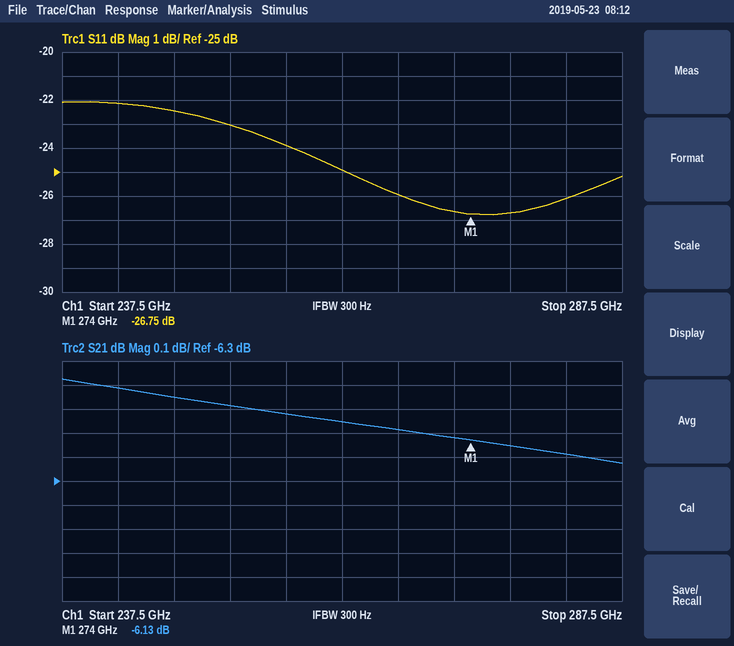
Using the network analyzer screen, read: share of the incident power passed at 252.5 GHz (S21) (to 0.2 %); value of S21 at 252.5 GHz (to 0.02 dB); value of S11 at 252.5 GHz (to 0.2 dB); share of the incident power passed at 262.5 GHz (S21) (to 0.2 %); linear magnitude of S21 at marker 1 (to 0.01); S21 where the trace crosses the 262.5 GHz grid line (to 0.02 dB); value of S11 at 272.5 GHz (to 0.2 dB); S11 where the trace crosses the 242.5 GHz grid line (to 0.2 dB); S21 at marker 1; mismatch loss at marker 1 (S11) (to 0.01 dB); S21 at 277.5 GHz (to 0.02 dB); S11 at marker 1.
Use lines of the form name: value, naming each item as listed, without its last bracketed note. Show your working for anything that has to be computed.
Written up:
share of the incident power passed at 252.5 GHz (S21): 10^(-5.98/10) ≈ 25.2 %
value of S21 at 252.5 GHz: -5.98 dB
value of S11 at 252.5 GHz: -23.0 dB
share of the incident power passed at 262.5 GHz (S21): 10^(-6.06/10) ≈ 24.8 %
linear magnitude of S21 at marker 1: 10^(-6.13/20) ≈ 0.49
S21 where the trace crosses the 262.5 GHz grid line: -6.06 dB
value of S11 at 272.5 GHz: -26.6 dB
S11 where the trace crosses the 242.5 GHz grid line: -22.2 dB
S21 at marker 1: -6.13 dB
mismatch loss at marker 1 (S11): −10 log10(1 − 10^(-26.75/10)) ≈ 0.01 dB
S21 at 277.5 GHz: -6.16 dB
S11 at marker 1: -26.75 dB
